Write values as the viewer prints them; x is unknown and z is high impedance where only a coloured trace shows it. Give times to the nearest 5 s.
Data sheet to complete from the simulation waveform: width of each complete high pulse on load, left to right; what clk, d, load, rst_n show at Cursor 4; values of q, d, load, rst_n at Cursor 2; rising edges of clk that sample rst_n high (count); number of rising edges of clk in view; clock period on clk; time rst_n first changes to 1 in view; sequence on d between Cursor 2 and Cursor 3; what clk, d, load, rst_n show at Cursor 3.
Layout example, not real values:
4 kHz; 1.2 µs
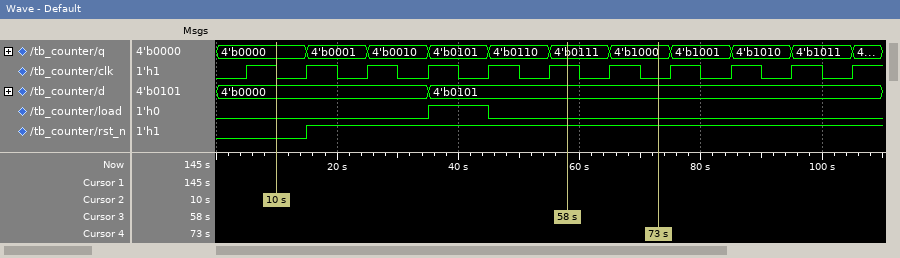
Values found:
10 s; clk=0, d=4'b0101, load=0, rst_n=1; q=4'b0000, d=4'b0000, load=0, rst_n=0; 9; 11; 10 s; 15 s; 4'b0000, 4'b0101; clk=1, d=4'b0101, load=0, rst_n=1
